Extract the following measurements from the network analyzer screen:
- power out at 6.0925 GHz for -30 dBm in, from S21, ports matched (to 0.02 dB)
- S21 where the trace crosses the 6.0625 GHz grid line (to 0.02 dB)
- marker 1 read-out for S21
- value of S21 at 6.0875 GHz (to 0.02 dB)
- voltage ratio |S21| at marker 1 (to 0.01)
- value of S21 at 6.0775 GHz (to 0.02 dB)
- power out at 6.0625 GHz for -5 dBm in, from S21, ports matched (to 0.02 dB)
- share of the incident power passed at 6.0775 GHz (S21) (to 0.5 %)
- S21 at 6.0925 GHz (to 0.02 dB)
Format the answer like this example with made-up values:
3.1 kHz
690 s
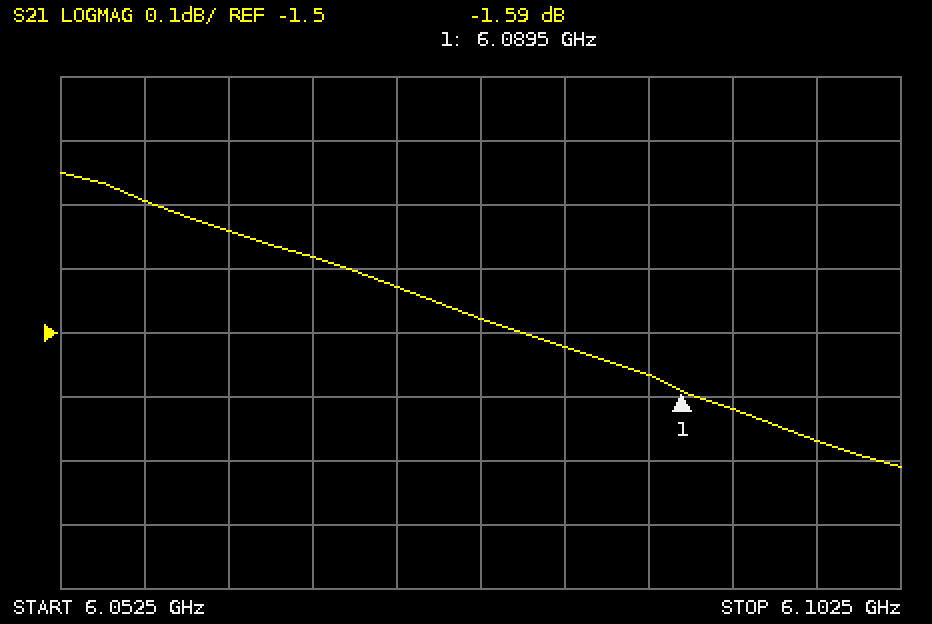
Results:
-31.62 dBm
-1.34 dB
-1.59 dB
-1.56 dB
0.83
-1.48 dB
-6.34 dBm
71.0 %
-1.62 dB
